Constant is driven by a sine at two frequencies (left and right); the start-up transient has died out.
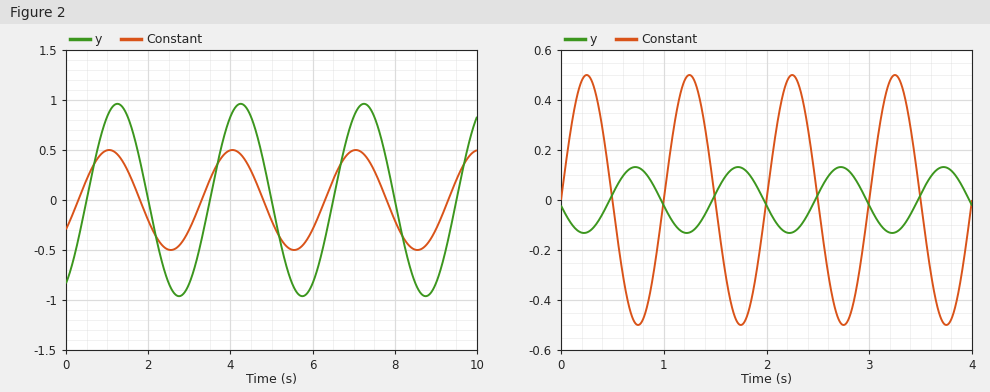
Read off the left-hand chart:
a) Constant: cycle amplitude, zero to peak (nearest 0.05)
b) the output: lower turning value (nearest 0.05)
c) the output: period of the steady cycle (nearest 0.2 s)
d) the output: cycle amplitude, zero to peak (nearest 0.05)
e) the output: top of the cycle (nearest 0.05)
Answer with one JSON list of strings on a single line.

["0.50", "-0.95", "3.0 s", "0.95", "0.95"]
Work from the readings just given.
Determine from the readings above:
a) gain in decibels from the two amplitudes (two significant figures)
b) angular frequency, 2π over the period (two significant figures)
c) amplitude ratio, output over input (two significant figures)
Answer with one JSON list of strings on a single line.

["5.6 dB", "2.1 rad/s", "1.9"]
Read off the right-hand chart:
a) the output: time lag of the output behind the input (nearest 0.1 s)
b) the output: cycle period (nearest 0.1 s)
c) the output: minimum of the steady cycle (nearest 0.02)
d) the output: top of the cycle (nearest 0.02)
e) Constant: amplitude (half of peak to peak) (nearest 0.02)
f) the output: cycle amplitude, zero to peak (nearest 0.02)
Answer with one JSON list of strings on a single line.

["0.5 s", "1.0 s", "-0.14", "0.14", "0.50", "0.14"]
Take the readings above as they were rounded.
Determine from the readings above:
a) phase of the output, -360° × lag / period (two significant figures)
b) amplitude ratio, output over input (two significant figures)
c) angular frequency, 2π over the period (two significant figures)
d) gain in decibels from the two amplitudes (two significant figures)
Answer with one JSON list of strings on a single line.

["-180°", "0.28", "6.3 rad/s", "-11 dB"]
